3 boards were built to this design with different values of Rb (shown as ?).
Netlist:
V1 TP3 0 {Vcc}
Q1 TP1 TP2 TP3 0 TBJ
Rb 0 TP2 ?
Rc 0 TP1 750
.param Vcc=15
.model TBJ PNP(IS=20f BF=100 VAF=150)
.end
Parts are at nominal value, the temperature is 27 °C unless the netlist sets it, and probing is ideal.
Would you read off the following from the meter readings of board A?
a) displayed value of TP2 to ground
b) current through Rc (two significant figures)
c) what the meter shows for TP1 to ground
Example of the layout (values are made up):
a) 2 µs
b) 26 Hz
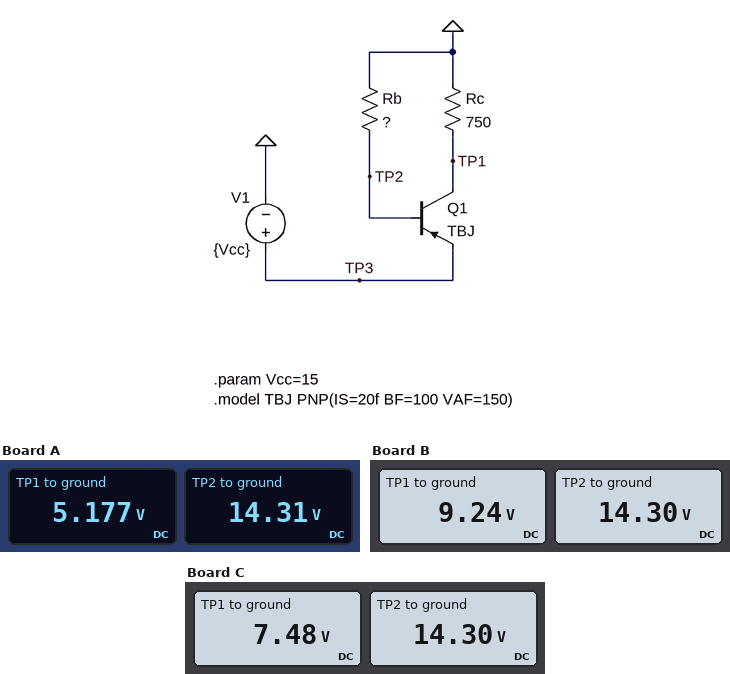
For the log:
a) 14.31 V
b) 6.9 mA
c) 5.177 V
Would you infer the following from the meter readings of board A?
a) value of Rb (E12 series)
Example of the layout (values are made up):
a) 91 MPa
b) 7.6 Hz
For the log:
a) 220 kΩ
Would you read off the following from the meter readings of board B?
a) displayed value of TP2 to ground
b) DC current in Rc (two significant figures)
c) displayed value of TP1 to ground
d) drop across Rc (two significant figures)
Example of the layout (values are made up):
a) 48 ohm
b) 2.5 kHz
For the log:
a) 14.30 V
b) 12 mA
c) 9.24 V
d) 9.2 V
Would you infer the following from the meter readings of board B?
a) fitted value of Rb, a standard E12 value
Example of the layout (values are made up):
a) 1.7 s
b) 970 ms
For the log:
a) 120 kΩ
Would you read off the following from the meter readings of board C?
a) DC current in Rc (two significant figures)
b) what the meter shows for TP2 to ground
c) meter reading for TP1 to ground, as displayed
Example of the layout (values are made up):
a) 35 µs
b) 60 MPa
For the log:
a) 10 mA
b) 14.30 V
c) 7.48 V
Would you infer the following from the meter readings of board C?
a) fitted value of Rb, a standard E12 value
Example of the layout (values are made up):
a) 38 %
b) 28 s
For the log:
a) 150 kΩ
